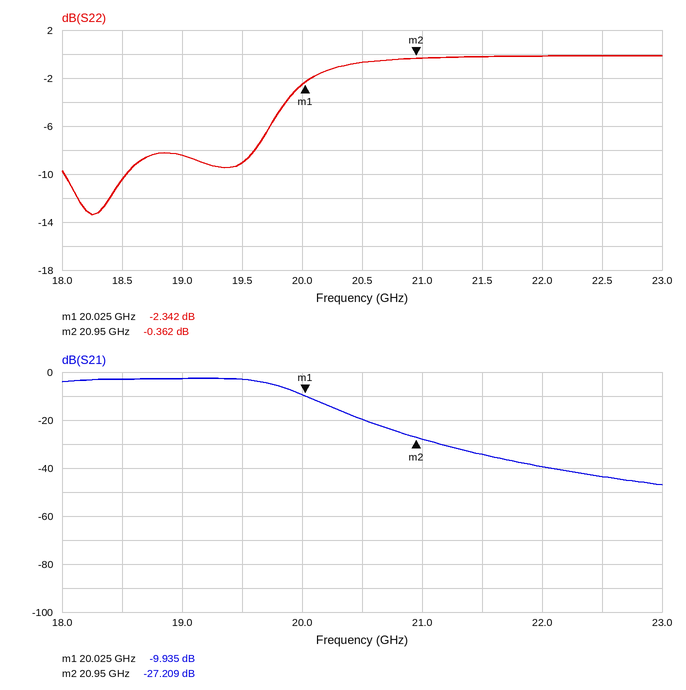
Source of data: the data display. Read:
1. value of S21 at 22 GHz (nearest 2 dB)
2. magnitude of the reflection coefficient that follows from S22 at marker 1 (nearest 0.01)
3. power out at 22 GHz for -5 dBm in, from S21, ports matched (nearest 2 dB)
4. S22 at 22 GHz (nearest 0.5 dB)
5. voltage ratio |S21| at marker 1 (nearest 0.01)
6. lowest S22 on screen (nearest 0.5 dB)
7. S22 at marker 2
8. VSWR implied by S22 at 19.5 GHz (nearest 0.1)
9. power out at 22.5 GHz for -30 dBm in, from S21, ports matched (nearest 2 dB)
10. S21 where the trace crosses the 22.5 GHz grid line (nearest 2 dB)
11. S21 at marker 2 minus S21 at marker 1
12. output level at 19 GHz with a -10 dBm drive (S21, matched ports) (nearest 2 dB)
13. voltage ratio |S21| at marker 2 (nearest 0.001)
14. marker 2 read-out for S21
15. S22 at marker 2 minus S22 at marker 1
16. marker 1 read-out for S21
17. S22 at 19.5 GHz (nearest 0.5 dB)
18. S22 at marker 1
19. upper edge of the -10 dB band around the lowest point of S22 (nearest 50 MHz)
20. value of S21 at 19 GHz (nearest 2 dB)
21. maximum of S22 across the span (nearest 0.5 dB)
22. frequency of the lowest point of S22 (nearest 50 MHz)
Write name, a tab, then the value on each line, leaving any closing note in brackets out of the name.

value of S21 at 22 GHz	-40 dB
magnitude of the reflection coefficient that follows from S22 at marker 1	0.76
power out at 22 GHz for -5 dBm in, from S21, ports matched	-44 dBm
S22 at 22 GHz	0.0 dB
voltage ratio |S21| at marker 1	0.32
lowest S22 on screen	-13.5 dB
S22 at marker 2	-0.362 dB
VSWR implied by S22 at 19.5 GHz	2.1
power out at 22.5 GHz for -30 dBm in, from S21, ports matched	-74 dBm
S21 where the trace crosses the 22.5 GHz grid line	-44 dB
S21 at marker 2 minus S21 at marker 1	-17.274 dB
output level at 19 GHz with a -10 dBm drive (S21, matched ports)	-12 dBm
voltage ratio |S21| at marker 2	0.044
marker 2 read-out for S21	-27.209 dB
S22 at marker 2 minus S22 at marker 1	1.980 dB
marker 1 read-out for S21	-9.935 dB
S22 at 19.5 GHz	-9.0 dB
S22 at marker 1	-2.342 dB
upper edge of the -10 dB band around the lowest point of S22	18.55 GHz
value of S21 at 19 GHz	-2 dB
maximum of S22 across the span	0.0 dB
frequency of the lowest point of S22	18.25 GHz
